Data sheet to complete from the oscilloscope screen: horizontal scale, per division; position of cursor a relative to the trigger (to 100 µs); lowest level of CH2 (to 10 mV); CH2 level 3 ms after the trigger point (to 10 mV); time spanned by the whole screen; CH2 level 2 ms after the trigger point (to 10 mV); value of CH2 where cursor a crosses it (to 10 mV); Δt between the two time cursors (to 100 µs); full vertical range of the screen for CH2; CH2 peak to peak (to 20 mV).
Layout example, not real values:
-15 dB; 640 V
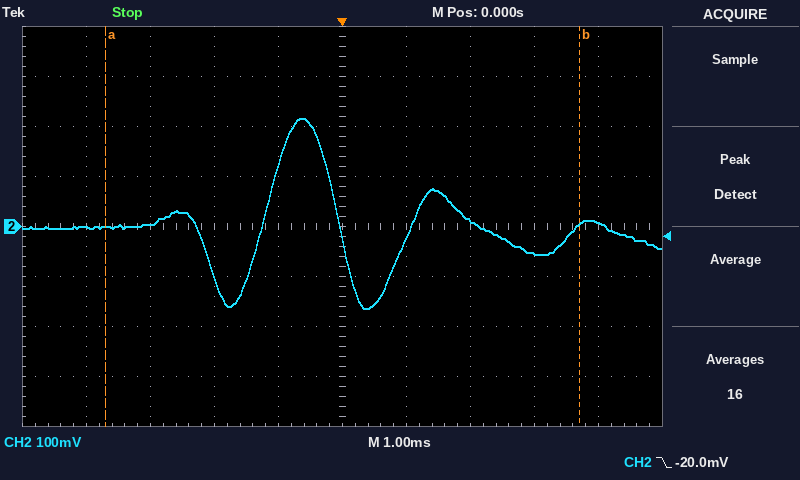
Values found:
1 ms; -3.7 ms; -160 mV; -50 mV; 10 ms; 10 mV; 0 mV; 7.4 ms; 800 mV; 380 mV
